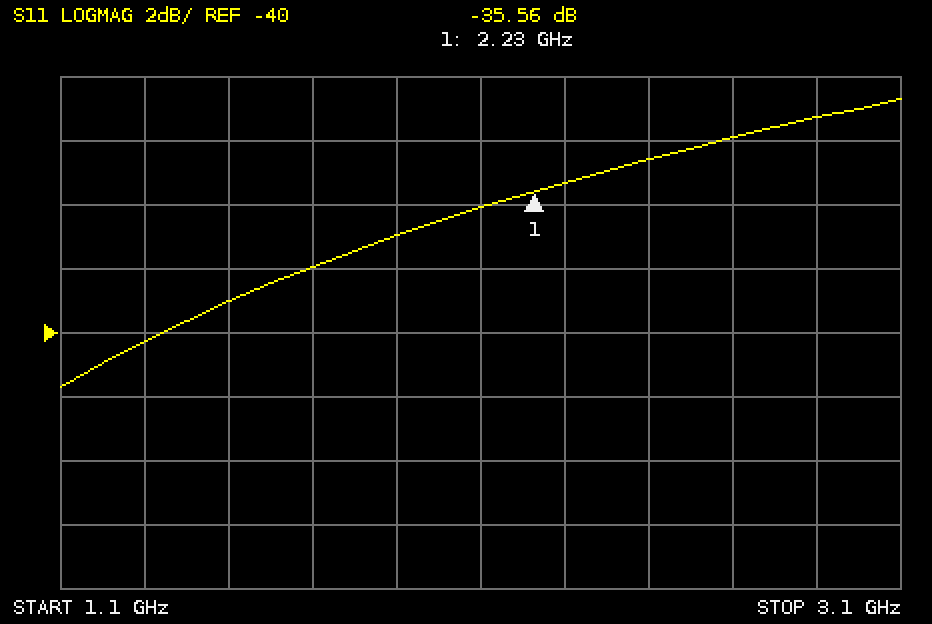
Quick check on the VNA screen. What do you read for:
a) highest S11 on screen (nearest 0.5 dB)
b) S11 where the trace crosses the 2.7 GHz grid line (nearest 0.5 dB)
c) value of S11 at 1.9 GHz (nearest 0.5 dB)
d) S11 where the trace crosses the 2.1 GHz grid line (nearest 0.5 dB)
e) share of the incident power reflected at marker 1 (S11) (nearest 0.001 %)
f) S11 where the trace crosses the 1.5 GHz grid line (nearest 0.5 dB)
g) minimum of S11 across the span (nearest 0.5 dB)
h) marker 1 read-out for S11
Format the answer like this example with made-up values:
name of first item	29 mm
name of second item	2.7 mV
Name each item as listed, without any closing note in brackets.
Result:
highest S11 on screen	-32.5 dB
S11 where the trace crosses the 2.7 GHz grid line	-34.0 dB
value of S11 at 1.9 GHz	-37.0 dB
S11 where the trace crosses the 2.1 GHz grid line	-36.0 dB
share of the incident power reflected at marker 1 (S11)	0.028 %
S11 where the trace crosses the 1.5 GHz grid line	-39.0 dB
minimum of S11 across the span	-41.5 dB
marker 1 read-out for S11	-35.56 dB
